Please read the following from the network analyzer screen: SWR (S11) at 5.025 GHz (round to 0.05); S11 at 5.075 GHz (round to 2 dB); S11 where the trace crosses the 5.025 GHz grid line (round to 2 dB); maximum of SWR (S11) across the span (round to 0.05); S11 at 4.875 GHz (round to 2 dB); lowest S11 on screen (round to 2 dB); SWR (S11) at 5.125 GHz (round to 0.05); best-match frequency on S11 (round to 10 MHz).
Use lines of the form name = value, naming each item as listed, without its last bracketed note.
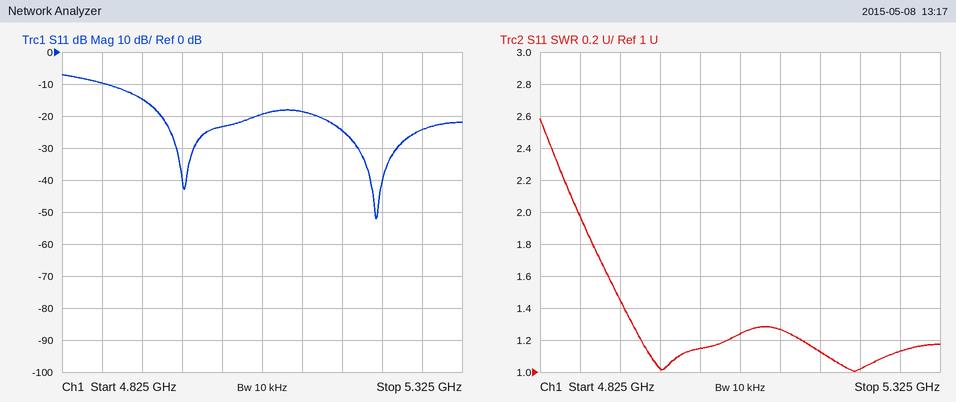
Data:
SWR (S11) at 5.025 GHz = 1.15
S11 at 5.075 GHz = -20 dB
S11 where the trace crosses the 5.025 GHz grid line = -24 dB
maximum of SWR (S11) across the span = 2.60
S11 at 4.875 GHz = -10 dB
lowest S11 on screen = -52 dB
SWR (S11) at 5.125 GHz = 1.25
best-match frequency on S11 = 5.22 GHz
